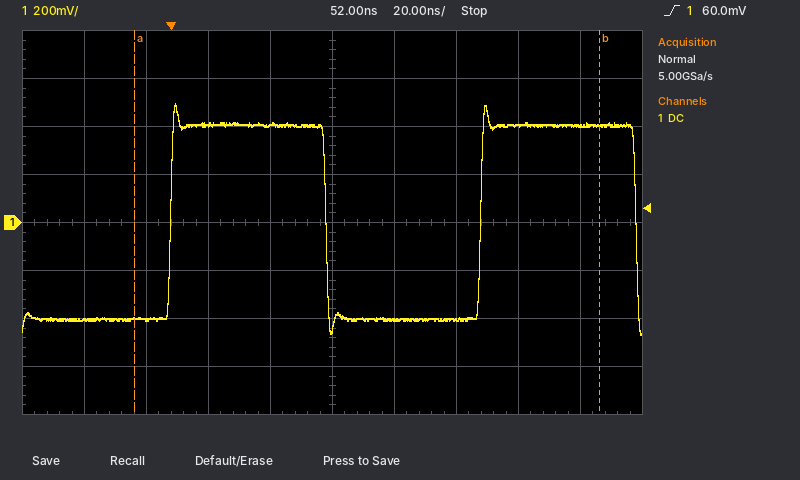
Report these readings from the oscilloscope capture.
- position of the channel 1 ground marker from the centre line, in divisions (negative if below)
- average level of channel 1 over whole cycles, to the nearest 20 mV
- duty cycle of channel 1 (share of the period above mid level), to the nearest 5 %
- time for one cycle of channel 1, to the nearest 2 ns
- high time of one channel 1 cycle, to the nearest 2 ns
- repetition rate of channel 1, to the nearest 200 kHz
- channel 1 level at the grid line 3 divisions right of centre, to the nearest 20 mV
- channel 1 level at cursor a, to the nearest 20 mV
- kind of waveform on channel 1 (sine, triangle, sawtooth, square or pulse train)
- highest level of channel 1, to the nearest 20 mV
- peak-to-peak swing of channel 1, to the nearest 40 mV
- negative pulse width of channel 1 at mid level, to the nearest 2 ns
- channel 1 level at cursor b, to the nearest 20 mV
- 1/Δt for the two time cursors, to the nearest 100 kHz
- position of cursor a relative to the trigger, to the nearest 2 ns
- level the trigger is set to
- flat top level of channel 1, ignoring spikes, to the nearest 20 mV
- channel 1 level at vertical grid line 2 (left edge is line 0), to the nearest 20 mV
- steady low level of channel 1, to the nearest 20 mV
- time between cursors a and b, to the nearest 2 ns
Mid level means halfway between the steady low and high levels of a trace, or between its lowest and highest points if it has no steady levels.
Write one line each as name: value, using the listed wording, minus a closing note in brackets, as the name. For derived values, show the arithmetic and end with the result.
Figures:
position of the channel 1 ground marker from the centre line, in divisions: 0.0 div
average level of channel 1 over whole cycles, to the nearest 20 mV: -400 mV + 0.5 × (400 mV − (-400 mV)) ≈ 0 mV
duty cycle of channel 1 (share of the period above mid level), to the nearest 5 %: 50 ns / 100 ns ≈ 50 %
time for one cycle of channel 1, to the nearest 2 ns: 100 ns
high time of one channel 1 cycle, to the nearest 2 ns: 50 ns
repetition rate of channel 1, to the nearest 200 kHz: 1 / 100 ns ≈ 10.0 MHz
channel 1 level at the grid line 3 divisions right of centre, to the nearest 20 mV: 400 mV
channel 1 level at cursor a, to the nearest 20 mV: -400 mV
kind of waveform on channel 1: square
highest level of channel 1, to the nearest 20 mV: 500 mV
peak-to-peak swing of channel 1, to the nearest 40 mV: 960 mV
negative pulse width of channel 1 at mid level, to the nearest 2 ns: 50 ns
channel 1 level at cursor b, to the nearest 20 mV: 400 mV
1/Δt for the two time cursors, to the nearest 100 kHz: 1 / 150 ns ≈ 6.7 MHz
position of cursor a relative to the trigger, to the nearest 2 ns: -12 ns
level the trigger is set to: 60.0 mV
flat top level of channel 1, ignoring spikes, to the nearest 20 mV: 400 mV
channel 1 level at vertical grid line 2 (left edge is line 0), to the nearest 20 mV: -400 mV
steady low level of channel 1, to the nearest 20 mV: -400 mV
time between cursors a and b, to the nearest 2 ns: 150 ns
